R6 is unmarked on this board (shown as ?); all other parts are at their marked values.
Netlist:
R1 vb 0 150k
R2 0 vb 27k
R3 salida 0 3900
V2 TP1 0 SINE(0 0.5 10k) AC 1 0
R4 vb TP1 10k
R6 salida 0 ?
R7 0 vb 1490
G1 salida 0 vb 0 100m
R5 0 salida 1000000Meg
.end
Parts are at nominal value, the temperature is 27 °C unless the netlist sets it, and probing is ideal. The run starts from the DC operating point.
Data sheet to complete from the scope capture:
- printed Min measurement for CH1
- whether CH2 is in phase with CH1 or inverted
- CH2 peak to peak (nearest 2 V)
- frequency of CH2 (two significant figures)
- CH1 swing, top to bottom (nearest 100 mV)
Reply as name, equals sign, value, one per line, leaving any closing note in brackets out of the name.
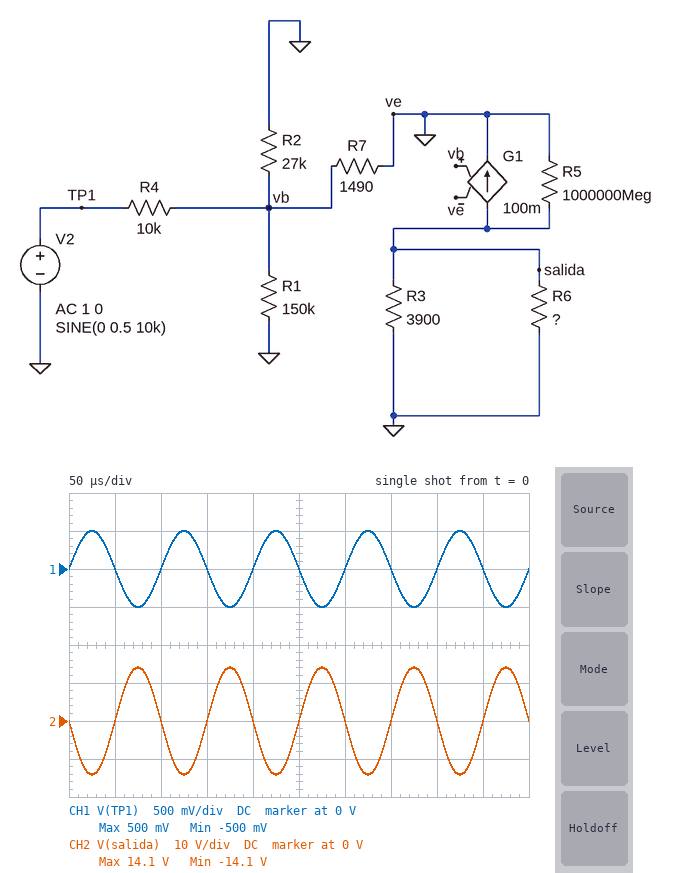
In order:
printed Min measurement for CH1 = -500 mV
whether CH2 is in phase with CH1 or inverted = inverted
CH2 peak to peak = 28 V
frequency of CH2 = 10 kHz
CH1 swing, top to bottom = 1.0 V
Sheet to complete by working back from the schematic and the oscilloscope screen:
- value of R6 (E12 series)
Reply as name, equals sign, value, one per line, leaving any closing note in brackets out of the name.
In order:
value of R6 = 5.6 kΩ
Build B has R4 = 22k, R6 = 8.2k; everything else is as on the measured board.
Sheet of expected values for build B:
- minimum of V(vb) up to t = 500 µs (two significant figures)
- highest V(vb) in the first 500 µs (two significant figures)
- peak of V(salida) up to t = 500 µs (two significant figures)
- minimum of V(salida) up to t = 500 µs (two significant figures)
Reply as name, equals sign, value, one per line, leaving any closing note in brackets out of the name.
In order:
minimum of V(vb) up to t = 500 µs = -30 mV
highest V(vb) in the first 500 µs = 30 mV
peak of V(salida) up to t = 500 µs = 7.9 V
minimum of V(salida) up to t = 500 µs = -7.9 V
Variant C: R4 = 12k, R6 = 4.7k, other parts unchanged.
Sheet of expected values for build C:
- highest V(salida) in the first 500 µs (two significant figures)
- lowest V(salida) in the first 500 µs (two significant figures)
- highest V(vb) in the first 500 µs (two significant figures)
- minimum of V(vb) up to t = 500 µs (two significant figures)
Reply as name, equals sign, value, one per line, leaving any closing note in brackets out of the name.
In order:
highest V(salida) in the first 500 µs = 11 V
lowest V(salida) in the first 500 µs = -11 V
highest V(vb) in the first 500 µs = 52 mV
minimum of V(vb) up to t = 500 µs = -52 mV
